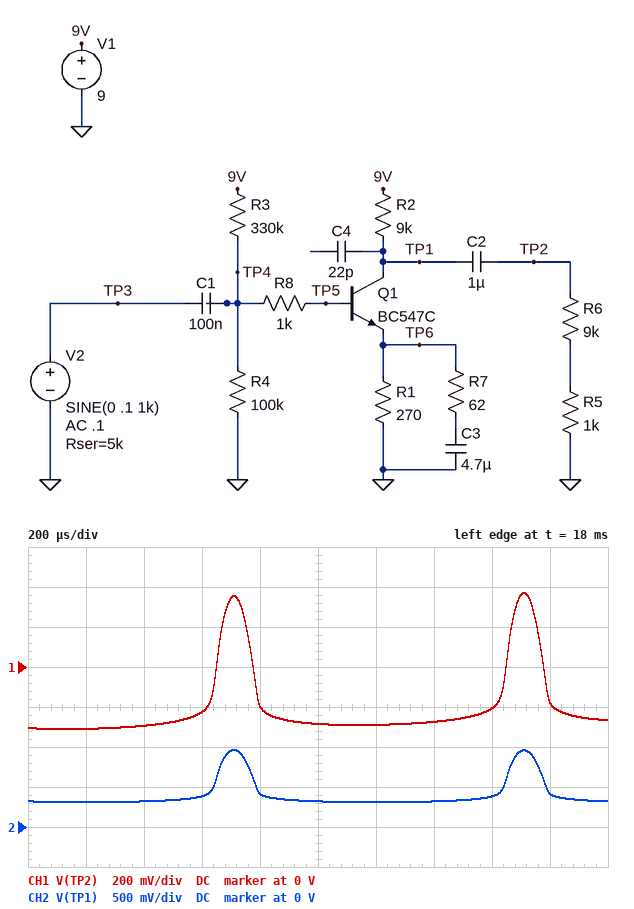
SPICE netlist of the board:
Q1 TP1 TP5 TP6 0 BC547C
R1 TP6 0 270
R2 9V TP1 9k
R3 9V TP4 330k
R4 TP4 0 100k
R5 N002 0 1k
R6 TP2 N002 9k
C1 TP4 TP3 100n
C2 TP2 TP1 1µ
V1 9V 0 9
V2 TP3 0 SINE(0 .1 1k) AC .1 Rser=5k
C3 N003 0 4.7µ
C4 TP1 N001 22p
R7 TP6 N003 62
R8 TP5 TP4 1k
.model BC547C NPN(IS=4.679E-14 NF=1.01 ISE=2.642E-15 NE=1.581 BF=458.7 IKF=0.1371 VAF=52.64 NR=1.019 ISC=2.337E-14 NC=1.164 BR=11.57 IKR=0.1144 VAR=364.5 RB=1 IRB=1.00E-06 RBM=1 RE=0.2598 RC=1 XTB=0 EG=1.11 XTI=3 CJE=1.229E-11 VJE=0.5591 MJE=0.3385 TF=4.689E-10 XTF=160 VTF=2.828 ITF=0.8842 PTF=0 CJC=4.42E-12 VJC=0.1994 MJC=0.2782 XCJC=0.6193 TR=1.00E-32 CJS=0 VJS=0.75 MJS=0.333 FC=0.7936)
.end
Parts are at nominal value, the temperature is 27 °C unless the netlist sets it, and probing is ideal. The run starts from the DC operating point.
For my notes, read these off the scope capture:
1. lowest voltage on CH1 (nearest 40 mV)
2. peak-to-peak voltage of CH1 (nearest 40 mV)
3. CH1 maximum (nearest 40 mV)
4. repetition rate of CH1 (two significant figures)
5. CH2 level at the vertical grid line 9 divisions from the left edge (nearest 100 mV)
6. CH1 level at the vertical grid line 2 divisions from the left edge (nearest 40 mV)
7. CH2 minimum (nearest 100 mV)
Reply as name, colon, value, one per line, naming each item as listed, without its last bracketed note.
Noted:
lowest voltage on CH1: -320 mV
peak-to-peak voltage of CH1: 680 mV
CH1 maximum: 360 mV
repetition rate of CH1: 1.0 kHz
CH2 level at the vertical grid line 9 divisions from the left edge: 400 mV
CH1 level at the vertical grid line 2 divisions from the left edge: -280 mV
CH2 minimum: 300 mV
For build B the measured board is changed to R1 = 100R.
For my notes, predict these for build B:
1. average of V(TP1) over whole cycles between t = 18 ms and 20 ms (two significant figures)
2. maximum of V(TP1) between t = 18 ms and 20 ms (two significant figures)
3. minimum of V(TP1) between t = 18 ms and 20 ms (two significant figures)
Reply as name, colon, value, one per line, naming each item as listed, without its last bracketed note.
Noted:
average of V(TP1) over whole cycles between t = 18 ms and 20 ms: 170 mV
maximum of V(TP1) between t = 18 ms and 20 ms: 260 mV
minimum of V(TP1) between t = 18 ms and 20 ms: 140 mV
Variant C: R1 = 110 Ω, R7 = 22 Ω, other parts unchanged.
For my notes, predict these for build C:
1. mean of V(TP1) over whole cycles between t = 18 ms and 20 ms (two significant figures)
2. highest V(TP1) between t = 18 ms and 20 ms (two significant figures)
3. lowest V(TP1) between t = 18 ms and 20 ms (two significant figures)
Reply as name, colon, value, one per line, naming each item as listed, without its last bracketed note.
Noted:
mean of V(TP1) over whole cycles between t = 18 ms and 20 ms: 180 mV
highest V(TP1) between t = 18 ms and 20 ms: 290 mV
lowest V(TP1) between t = 18 ms and 20 ms: 150 mV
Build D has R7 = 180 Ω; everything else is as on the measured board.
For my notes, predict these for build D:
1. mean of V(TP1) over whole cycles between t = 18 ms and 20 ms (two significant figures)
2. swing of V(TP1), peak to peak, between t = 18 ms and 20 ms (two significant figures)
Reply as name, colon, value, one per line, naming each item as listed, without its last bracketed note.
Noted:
mean of V(TP1) over whole cycles between t = 18 ms and 20 ms: 380 mV
swing of V(TP1), peak to peak, between t = 18 ms and 20 ms: 400 mV
